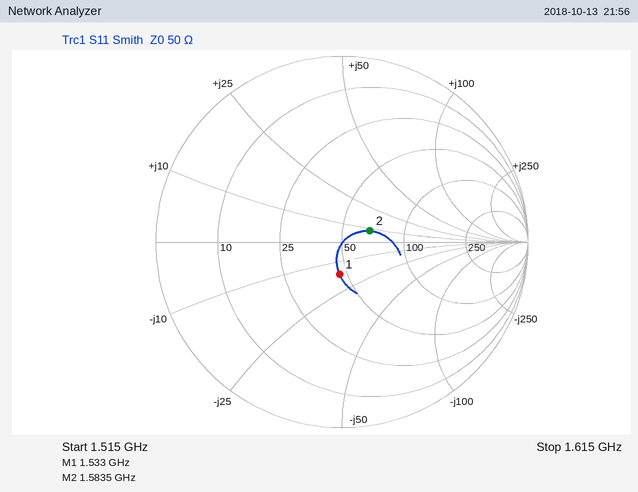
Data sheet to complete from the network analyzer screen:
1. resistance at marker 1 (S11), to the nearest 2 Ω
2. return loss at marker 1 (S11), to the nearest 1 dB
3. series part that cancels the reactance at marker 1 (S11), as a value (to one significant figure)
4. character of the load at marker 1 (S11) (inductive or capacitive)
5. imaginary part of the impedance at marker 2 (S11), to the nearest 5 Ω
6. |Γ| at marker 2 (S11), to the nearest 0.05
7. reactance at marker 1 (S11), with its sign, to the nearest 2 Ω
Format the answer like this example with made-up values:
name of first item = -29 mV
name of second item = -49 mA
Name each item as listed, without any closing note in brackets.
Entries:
resistance at marker 1 (S11), to the nearest 2 Ω = 46 Ω
return loss at marker 1 (S11), to the nearest 1 dB = 15 dB
series part that cancels the reactance at marker 1 (S11), as a value = 2 nH
character of the load at marker 1 (S11) = capacitive
imaginary part of the impedance at marker 2 (S11), to the nearest 5 Ω = +10 Ω
|Γ| at marker 2 (S11), to the nearest 0.05 = 0.15
reactance at marker 1 (S11), with its sign, to the nearest 2 Ω = -16 Ω
